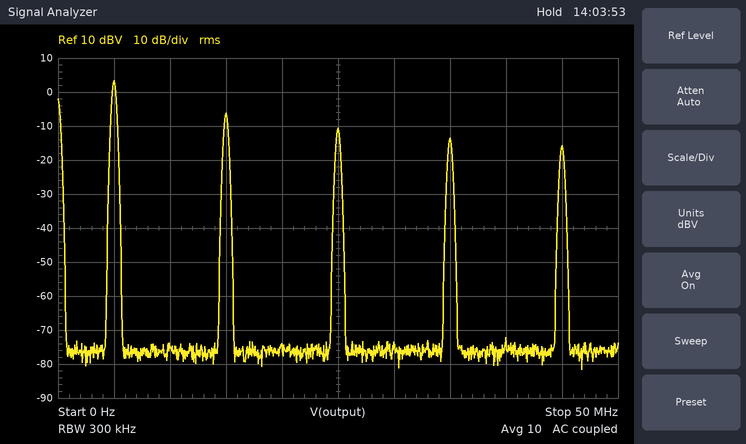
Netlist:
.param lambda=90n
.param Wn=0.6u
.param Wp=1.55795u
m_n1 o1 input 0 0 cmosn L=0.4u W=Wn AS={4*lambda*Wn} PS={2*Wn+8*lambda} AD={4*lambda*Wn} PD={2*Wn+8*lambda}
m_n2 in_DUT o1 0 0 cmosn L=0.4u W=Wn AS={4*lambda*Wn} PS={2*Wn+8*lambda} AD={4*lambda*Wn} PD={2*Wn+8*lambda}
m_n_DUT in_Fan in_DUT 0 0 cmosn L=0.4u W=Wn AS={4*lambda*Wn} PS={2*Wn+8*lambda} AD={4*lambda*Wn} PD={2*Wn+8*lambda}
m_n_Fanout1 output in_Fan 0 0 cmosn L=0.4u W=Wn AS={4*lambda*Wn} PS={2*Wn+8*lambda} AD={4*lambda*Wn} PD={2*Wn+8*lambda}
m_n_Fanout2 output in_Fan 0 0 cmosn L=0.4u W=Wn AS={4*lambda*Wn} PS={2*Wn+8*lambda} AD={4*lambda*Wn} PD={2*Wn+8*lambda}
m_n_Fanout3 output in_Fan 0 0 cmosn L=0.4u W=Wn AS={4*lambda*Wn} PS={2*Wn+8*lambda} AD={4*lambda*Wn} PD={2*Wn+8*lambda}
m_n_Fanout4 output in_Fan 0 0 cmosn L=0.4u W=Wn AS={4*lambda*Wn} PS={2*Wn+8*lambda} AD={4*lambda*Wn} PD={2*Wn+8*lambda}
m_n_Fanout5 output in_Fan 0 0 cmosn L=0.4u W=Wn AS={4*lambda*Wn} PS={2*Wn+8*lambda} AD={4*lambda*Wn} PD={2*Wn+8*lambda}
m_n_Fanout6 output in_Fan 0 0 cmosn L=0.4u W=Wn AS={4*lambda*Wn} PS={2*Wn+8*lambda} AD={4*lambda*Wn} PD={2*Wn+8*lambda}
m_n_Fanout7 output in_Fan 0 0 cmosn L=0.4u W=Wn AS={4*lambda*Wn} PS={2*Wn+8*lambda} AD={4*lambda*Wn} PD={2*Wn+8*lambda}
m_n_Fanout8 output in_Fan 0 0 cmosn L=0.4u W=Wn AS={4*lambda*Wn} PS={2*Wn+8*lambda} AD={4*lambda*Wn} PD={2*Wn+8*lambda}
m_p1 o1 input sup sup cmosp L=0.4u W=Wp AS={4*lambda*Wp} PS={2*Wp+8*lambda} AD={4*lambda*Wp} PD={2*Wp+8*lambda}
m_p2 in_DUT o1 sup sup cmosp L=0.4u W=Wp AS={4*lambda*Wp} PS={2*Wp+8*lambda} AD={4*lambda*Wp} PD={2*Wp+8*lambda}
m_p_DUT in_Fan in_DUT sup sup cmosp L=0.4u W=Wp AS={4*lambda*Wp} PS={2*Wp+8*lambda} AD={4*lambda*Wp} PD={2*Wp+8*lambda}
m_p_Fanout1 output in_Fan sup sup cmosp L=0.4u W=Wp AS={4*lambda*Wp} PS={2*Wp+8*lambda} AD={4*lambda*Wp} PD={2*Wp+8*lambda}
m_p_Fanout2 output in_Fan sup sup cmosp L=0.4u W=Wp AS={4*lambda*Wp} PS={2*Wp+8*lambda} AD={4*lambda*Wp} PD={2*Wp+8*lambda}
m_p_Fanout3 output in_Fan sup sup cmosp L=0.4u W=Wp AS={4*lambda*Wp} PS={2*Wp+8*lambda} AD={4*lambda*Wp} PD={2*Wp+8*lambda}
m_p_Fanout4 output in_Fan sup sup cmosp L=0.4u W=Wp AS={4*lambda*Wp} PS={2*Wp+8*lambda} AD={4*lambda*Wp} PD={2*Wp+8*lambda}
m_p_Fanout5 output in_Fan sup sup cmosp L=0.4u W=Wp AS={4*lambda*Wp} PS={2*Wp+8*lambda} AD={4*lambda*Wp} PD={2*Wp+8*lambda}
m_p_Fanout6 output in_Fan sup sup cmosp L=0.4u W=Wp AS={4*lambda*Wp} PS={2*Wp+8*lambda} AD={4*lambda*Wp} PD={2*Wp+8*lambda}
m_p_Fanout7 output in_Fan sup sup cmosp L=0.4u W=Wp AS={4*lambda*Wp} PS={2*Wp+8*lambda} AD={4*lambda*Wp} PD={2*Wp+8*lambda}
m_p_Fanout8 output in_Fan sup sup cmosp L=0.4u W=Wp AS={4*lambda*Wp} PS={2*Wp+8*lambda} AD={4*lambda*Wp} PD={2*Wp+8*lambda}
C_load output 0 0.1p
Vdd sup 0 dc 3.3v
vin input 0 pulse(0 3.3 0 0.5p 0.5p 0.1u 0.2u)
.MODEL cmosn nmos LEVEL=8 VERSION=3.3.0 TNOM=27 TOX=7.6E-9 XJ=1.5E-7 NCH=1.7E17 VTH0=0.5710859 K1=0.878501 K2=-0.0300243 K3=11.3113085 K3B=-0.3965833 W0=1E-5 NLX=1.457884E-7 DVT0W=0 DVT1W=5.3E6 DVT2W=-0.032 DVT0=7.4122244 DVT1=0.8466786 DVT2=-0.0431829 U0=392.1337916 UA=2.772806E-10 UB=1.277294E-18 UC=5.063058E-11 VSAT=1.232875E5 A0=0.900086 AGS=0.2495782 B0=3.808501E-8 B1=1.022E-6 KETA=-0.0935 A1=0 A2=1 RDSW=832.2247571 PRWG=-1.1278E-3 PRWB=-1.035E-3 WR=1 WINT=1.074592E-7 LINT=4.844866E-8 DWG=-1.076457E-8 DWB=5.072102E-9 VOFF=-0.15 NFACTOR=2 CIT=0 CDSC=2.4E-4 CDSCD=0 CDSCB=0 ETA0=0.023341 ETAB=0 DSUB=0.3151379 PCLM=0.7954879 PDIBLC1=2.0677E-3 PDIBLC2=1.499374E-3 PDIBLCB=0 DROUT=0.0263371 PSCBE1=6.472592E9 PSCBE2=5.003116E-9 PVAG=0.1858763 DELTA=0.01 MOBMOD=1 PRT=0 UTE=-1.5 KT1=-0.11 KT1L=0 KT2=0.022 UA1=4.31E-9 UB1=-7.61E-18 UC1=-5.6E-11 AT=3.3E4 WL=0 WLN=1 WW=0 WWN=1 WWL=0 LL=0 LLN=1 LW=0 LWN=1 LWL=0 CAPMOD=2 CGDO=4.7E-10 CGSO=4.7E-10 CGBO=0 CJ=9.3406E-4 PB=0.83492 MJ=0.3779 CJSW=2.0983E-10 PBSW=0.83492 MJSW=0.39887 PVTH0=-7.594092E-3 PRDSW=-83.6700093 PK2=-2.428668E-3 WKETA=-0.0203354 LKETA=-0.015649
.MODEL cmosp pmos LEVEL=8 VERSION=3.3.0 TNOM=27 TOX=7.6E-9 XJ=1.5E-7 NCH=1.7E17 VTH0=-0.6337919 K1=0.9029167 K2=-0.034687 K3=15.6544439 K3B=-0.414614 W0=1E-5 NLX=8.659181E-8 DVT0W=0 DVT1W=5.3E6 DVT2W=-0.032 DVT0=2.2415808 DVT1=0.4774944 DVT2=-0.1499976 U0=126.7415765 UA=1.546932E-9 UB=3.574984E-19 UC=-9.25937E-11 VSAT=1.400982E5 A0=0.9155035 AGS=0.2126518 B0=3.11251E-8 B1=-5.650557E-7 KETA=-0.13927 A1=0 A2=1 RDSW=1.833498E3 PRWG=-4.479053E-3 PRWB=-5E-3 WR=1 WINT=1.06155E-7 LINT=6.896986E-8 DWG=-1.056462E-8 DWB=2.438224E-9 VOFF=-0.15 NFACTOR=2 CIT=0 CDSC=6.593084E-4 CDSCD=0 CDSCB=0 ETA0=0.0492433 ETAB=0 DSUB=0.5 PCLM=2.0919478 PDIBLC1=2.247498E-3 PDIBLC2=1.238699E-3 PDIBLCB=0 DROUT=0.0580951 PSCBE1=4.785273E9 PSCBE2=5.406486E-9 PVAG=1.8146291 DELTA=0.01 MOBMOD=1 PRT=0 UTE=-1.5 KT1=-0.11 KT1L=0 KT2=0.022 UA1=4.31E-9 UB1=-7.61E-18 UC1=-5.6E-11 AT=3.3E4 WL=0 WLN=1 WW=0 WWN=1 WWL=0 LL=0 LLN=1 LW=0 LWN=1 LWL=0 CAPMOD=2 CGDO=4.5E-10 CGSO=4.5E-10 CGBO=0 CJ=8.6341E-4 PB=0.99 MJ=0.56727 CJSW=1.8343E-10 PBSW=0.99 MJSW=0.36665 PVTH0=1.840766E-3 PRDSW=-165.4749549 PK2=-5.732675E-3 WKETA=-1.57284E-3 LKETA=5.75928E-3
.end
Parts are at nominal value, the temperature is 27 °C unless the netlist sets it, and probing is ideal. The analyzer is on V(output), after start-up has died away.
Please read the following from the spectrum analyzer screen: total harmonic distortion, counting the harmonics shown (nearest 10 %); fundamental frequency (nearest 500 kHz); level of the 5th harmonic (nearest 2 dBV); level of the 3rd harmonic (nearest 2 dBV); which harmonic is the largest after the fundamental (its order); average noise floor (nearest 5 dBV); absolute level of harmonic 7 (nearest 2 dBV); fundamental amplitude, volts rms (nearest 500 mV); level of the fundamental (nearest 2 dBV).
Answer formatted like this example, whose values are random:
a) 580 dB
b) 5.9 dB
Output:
a) 40 %
b) 5.0 MHz
c) -10 dBV
d) -6 dBV
e) 3
f) -75 dBV
g) -14 dBV
h) 1.5 V
i) 4 dBV
